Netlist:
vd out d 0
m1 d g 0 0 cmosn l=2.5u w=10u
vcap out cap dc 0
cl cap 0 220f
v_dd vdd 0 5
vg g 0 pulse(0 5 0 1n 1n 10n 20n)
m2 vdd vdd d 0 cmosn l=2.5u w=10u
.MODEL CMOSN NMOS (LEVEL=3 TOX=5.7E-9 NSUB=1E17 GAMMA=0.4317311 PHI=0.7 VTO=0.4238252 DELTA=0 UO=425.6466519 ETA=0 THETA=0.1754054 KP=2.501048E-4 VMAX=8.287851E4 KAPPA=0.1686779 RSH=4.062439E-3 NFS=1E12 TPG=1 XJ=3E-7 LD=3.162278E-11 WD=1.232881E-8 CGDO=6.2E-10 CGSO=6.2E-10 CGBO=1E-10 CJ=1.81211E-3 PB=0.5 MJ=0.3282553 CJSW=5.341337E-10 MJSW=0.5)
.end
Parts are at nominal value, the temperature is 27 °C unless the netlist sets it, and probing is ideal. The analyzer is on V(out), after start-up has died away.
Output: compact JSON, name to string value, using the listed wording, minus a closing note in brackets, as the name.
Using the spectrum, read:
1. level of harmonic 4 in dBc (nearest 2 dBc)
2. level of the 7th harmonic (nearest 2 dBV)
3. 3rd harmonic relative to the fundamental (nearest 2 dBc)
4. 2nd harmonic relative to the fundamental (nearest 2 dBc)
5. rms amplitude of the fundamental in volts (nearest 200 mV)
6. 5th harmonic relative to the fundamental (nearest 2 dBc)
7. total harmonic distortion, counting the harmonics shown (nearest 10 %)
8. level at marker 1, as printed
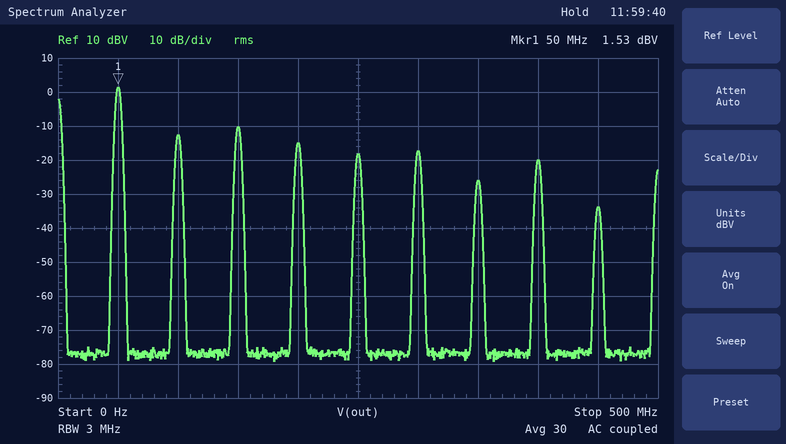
{"level of harmonic 4 in dBc": "-16 dBc", "level of the 7th harmonic": "-26 dBV", "3rd harmonic relative to the fundamental": "-12 dBc", "2nd harmonic relative to the fundamental": "-14 dBc", "rms amplitude of the fundamental in volts": "1.2 V", "5th harmonic relative to the fundamental": "-20 dBc", "total harmonic distortion, counting the harmonics shown": "40 %", "level at marker 1, as printed": "1.53 dBV"}
